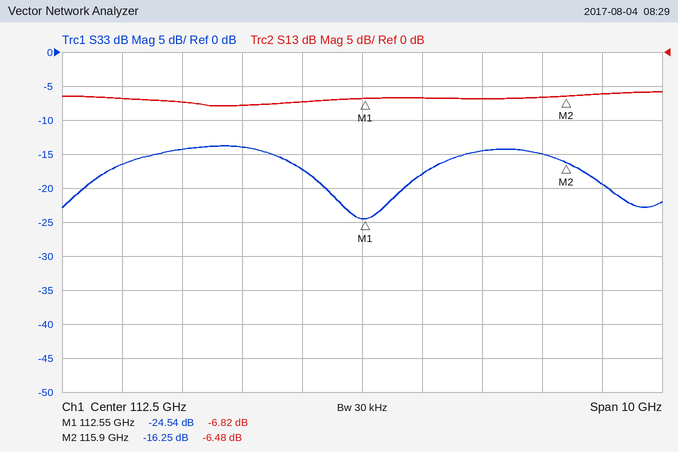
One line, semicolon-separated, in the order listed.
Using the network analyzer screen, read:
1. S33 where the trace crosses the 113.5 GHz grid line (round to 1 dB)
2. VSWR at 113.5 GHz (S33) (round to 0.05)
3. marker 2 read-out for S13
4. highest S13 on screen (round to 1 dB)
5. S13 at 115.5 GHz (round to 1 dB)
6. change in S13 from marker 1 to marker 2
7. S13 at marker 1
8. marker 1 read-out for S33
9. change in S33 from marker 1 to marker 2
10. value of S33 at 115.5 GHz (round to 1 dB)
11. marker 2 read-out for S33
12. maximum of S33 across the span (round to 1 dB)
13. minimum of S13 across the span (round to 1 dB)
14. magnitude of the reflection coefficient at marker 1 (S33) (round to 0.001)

-18 dB; 1.30; -6.48 dB; -6 dB; -7 dB; 0.34 dB; -6.82 dB; -24.54 dB; 8.29 dB; -15 dB; -16.25 dB; -14 dB; -8 dB; 0.059
